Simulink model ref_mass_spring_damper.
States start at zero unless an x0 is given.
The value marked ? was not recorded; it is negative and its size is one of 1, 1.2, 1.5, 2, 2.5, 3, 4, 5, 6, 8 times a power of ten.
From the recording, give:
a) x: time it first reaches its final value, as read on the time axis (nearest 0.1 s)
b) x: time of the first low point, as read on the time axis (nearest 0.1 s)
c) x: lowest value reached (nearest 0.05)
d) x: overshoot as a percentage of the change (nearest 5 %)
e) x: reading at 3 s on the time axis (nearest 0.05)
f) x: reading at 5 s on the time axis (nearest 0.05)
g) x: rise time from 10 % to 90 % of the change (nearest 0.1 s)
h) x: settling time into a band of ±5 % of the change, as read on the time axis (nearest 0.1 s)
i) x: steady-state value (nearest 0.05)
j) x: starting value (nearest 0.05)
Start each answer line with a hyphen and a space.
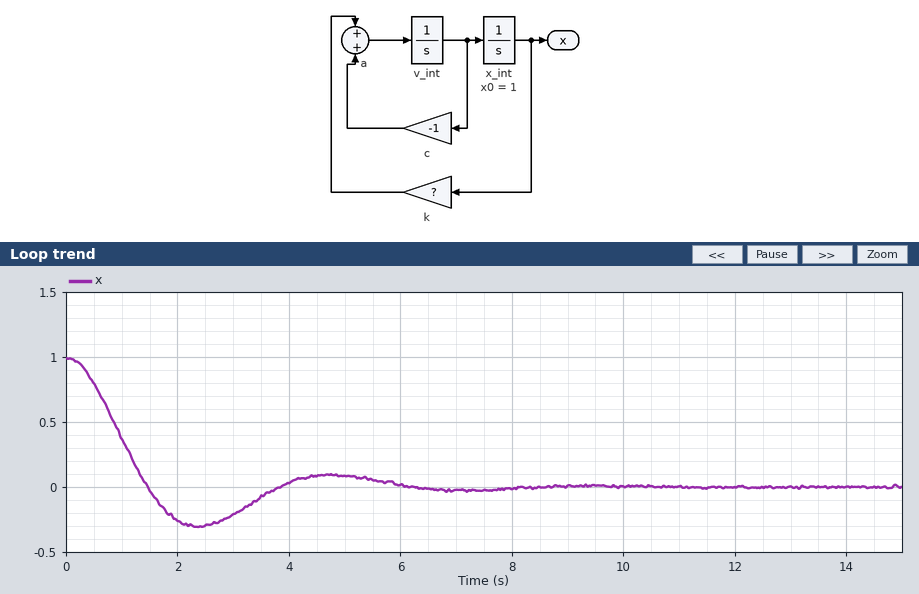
- 1.5 s
- 2.4 s
- -0.30
- 30 %
- -0.20
- 0.10
- 1.0 s
- 5.6 s
- 0.00
- 1.00
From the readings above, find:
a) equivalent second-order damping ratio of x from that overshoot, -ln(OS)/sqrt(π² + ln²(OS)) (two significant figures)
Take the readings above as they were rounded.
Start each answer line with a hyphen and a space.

- 0.36
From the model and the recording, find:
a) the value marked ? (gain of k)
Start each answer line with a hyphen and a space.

- -2
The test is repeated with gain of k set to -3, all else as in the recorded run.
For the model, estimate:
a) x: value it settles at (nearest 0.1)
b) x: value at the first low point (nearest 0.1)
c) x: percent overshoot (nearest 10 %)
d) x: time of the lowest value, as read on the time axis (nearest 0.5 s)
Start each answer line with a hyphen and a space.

- 0.0
- -0.4
- 40 %
- 2.0 s
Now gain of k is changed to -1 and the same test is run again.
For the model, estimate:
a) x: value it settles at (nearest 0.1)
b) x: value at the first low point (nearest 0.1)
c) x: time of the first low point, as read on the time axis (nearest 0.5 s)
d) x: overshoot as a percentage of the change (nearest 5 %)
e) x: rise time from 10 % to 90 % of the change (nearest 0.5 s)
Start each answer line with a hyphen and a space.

- 0.0
- -0.2
- 3.5 s
- 15 %
- 1.5 s
